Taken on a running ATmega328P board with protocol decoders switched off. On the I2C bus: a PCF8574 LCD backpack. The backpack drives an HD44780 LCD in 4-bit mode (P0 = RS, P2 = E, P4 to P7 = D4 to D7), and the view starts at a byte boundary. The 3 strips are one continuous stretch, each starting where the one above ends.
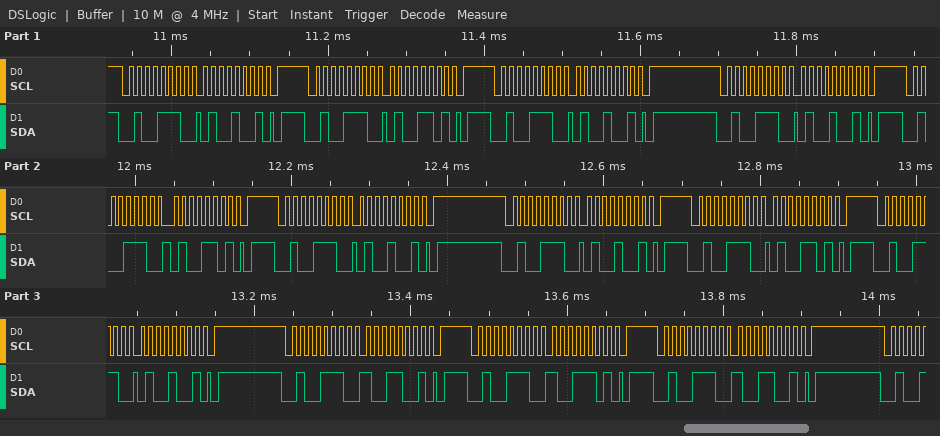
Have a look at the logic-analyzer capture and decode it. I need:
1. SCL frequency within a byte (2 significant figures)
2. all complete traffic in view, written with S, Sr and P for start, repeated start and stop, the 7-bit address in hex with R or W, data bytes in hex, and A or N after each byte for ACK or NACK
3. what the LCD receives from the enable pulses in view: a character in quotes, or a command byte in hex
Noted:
100 kHz
S 27W A 49 A P S 27W A 4D A P S 27W A 49 A P S 27W A 49 A P S 27W A 4D A P S 27W A 49 A P S 27W A 49 A P S 27W A 4D A P S 27W A 49 A P S 27W A 99 A P S 27W A 9D A P S 27W A 99 A P
'D' 'I'
